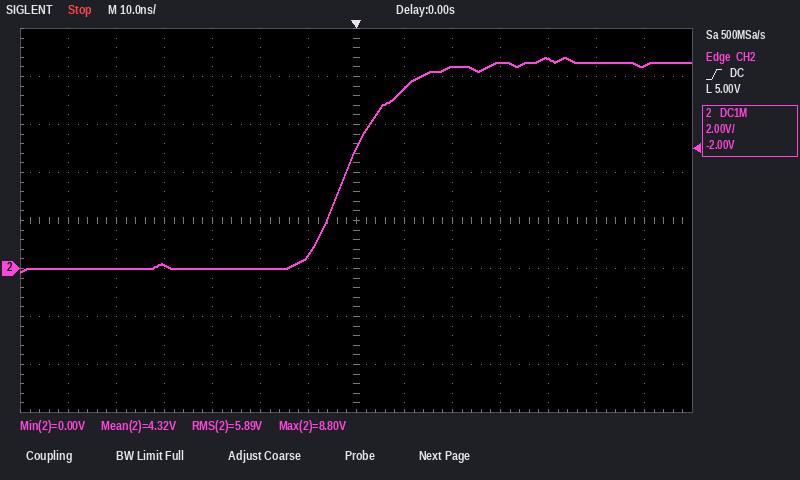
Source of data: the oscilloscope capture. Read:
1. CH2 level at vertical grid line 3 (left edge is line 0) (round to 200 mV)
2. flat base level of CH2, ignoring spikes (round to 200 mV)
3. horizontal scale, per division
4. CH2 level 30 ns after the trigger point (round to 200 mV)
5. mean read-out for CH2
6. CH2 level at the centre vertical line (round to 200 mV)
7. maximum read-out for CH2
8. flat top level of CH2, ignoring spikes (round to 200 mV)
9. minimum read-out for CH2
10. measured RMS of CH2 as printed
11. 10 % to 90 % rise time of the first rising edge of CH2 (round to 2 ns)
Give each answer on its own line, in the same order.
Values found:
200 mV
0.0 V
10 ns
8.6 V
4.32 V
5.0 V
8.80 V
8.6 V
0.00 V
5.89 V
20 ns
